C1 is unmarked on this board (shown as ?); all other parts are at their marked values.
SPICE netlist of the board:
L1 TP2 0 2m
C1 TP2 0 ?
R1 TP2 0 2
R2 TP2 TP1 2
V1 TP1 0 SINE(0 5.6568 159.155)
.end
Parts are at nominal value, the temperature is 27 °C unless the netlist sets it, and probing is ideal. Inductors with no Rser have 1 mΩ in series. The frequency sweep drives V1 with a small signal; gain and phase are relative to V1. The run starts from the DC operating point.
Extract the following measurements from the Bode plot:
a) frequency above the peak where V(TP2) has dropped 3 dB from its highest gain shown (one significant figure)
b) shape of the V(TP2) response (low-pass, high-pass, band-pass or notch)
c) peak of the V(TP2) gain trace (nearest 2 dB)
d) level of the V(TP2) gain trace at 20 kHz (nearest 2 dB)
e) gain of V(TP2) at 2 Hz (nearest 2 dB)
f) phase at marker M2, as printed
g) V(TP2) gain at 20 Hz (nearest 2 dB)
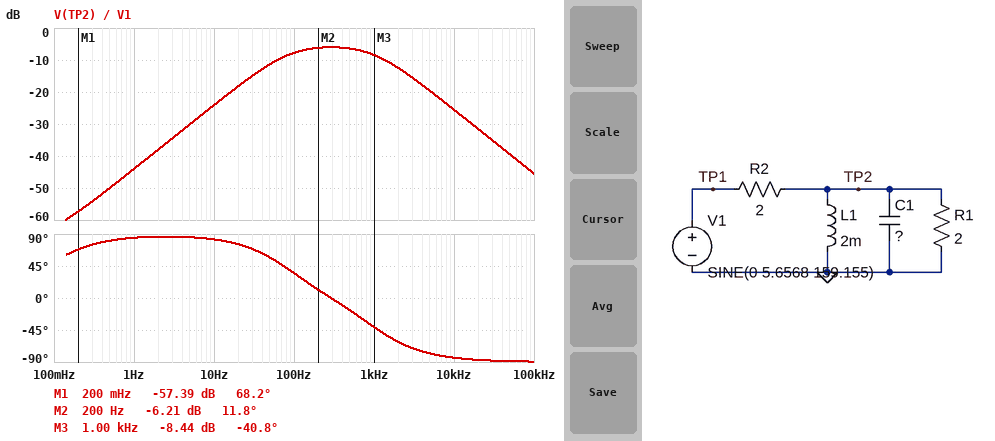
1 kHz
band-pass
-6 dB
-32 dB
-38 dB
11.8 deg
-18 dB
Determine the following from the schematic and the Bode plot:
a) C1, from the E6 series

150 µF
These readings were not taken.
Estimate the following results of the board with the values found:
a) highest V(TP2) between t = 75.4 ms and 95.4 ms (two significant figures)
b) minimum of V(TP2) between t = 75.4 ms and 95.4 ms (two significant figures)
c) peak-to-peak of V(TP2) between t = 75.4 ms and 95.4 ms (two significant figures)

2.7 V
-2.7 V
5.3 V
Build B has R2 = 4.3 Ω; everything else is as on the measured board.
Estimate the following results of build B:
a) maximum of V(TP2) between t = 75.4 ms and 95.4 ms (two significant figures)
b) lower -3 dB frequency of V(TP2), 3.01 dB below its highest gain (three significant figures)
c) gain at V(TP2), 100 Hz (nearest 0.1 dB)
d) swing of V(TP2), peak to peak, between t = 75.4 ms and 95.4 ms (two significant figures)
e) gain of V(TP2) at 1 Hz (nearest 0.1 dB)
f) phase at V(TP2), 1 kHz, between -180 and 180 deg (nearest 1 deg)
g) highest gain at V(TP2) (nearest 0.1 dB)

1.6 V
96.7 Hz
-12.8 dB
3.2 V
-50.7 dB
-50 deg
-10.0 dB
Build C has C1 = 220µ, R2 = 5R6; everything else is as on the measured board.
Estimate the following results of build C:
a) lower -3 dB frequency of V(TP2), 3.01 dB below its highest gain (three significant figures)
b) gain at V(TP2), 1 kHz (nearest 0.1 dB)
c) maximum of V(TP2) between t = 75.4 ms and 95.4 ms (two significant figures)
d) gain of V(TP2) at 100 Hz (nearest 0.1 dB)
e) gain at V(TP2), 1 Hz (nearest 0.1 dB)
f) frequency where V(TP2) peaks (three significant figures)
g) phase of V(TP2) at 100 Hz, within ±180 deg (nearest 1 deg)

97.8 Hz
-18.3 dB
1.4 V
-14.5 dB
-53.0 dB
240 Hz
44 deg
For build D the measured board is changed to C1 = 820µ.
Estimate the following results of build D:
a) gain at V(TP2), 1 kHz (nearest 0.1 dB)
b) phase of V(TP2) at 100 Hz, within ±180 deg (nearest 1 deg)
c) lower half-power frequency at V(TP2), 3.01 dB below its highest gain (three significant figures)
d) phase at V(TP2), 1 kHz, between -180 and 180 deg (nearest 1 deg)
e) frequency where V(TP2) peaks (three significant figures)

-20.3 dB
16 deg
60.7 Hz
-79 deg
124 Hz
